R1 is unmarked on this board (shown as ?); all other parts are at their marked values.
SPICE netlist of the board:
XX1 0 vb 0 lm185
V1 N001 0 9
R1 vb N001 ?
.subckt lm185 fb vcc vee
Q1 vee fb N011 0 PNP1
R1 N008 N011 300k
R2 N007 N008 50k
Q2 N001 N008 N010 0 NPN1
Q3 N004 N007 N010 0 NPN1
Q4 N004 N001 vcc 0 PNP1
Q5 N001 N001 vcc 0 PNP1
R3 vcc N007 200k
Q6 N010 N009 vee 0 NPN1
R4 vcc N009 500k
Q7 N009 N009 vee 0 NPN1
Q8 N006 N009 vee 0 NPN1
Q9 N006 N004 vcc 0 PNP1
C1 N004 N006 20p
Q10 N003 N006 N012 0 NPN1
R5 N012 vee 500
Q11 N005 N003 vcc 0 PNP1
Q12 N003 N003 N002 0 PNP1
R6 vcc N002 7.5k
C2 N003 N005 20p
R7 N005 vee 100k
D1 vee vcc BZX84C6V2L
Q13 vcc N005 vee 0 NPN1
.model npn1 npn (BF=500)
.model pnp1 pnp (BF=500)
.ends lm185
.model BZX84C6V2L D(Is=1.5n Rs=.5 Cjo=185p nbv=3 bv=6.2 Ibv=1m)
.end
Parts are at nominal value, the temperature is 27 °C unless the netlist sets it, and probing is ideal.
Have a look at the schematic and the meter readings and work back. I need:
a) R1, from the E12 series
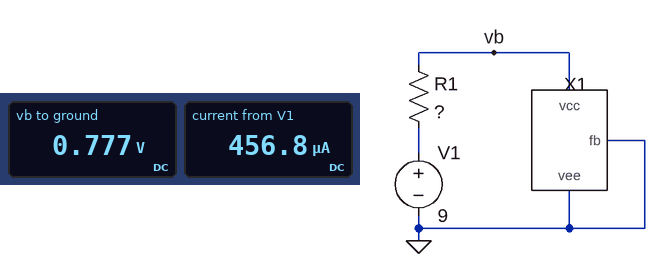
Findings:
18 kΩ
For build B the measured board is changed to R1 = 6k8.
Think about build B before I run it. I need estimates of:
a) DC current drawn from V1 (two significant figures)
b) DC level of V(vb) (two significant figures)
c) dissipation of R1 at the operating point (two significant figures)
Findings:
1.2 mA
800 mV
9.9 mW
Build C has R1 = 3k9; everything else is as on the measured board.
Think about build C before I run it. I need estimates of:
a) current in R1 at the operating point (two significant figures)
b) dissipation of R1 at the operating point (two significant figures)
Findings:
2.1 mA
17 mW
